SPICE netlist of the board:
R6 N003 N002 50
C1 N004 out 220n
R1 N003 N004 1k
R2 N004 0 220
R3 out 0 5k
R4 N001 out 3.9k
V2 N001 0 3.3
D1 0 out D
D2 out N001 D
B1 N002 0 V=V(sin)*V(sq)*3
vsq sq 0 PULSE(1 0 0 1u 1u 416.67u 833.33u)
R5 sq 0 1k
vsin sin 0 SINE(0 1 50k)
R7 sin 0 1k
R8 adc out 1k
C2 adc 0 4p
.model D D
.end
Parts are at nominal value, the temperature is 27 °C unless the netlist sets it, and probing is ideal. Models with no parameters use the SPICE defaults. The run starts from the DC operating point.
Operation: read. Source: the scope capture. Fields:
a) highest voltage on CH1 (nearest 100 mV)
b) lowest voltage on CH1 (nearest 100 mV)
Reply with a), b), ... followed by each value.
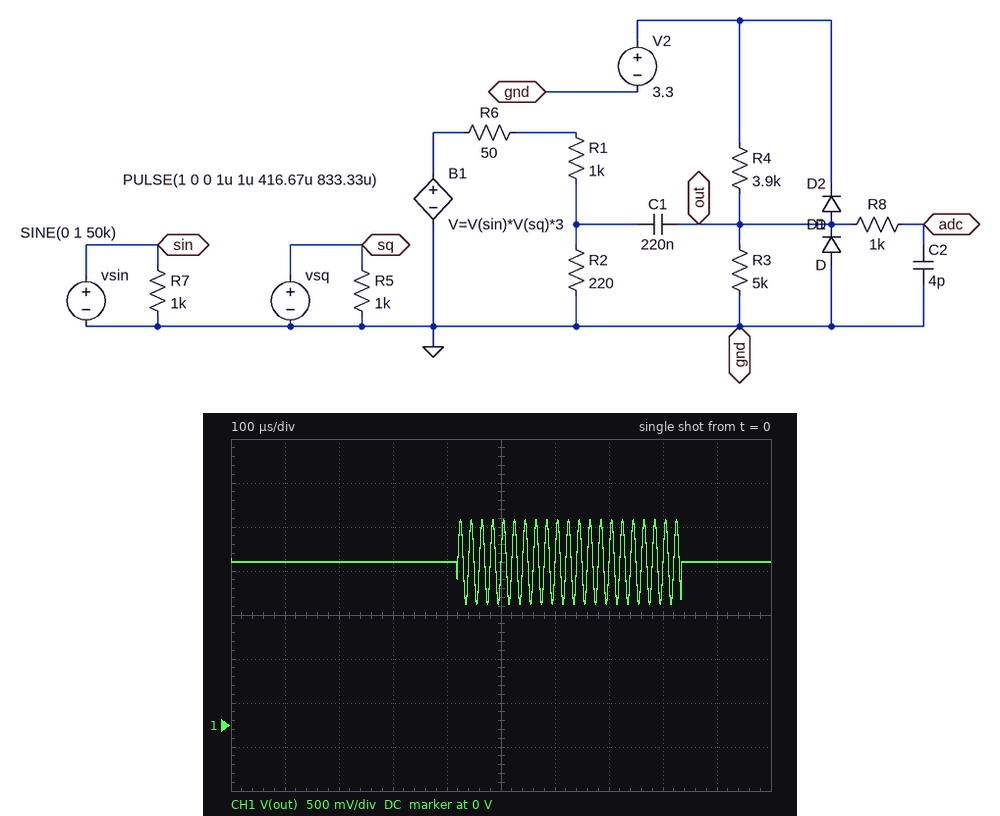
a) 2.3 V
b) 1.4 V
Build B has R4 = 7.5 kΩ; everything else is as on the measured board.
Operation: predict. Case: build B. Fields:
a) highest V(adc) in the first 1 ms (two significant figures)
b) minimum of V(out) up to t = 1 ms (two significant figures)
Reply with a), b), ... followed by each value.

a) 1.8 V
b) 830 mV
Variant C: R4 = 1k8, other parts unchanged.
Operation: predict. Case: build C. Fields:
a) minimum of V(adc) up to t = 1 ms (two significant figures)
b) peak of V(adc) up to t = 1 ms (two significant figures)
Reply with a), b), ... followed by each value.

a) 2.0 V
b) 2.9 V
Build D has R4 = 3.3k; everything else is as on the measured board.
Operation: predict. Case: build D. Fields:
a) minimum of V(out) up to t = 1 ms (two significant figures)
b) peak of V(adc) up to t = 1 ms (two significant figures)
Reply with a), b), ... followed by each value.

a) 1.5 V
b) 2.5 V
